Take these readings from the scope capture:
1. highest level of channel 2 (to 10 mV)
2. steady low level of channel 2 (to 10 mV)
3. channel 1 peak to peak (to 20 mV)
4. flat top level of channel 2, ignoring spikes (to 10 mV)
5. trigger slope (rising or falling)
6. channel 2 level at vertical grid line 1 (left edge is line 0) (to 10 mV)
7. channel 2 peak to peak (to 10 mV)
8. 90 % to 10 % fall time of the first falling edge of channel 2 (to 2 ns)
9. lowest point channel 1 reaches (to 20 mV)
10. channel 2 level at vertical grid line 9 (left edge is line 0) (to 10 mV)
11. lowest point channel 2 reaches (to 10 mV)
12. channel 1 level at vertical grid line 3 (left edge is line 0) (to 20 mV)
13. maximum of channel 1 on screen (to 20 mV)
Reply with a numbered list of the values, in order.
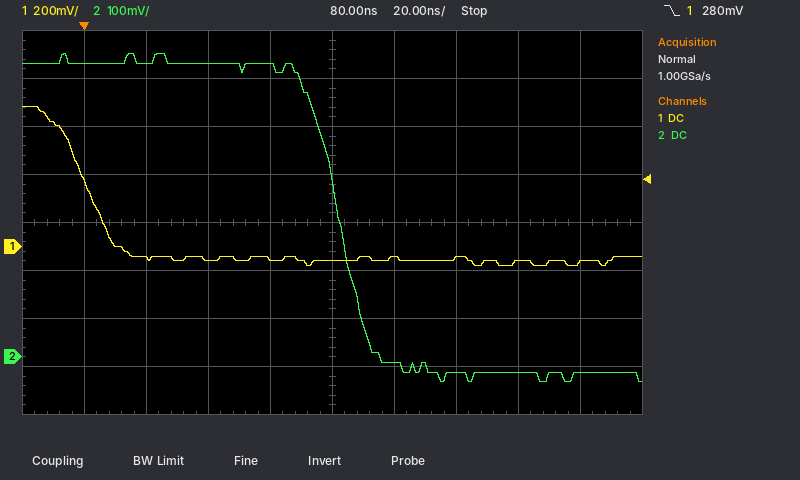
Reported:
1. 630 mV
2. -30 mV
3. 660 mV
4. 610 mV
5. falling
6. 610 mV
7. 680 mV
8. 20 ns
9. -80 mV
10. -30 mV
11. -50 mV
12. -60 mV
13. 580 mV
